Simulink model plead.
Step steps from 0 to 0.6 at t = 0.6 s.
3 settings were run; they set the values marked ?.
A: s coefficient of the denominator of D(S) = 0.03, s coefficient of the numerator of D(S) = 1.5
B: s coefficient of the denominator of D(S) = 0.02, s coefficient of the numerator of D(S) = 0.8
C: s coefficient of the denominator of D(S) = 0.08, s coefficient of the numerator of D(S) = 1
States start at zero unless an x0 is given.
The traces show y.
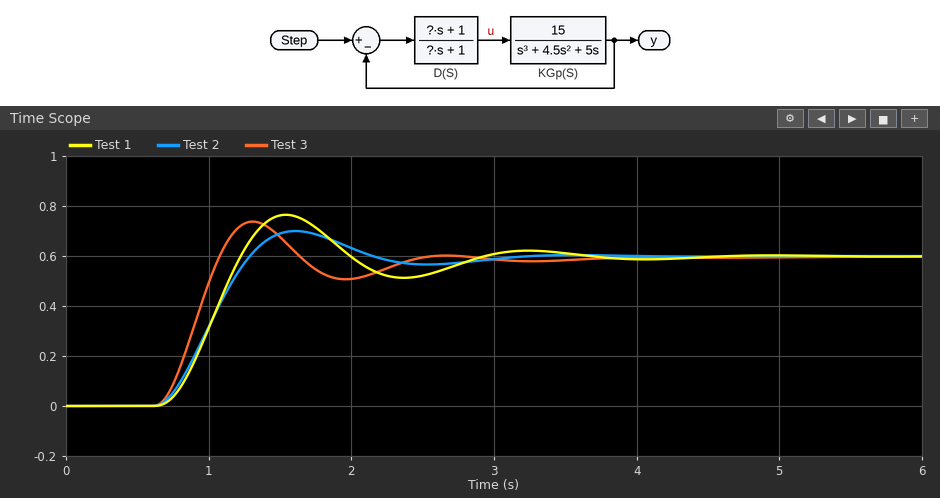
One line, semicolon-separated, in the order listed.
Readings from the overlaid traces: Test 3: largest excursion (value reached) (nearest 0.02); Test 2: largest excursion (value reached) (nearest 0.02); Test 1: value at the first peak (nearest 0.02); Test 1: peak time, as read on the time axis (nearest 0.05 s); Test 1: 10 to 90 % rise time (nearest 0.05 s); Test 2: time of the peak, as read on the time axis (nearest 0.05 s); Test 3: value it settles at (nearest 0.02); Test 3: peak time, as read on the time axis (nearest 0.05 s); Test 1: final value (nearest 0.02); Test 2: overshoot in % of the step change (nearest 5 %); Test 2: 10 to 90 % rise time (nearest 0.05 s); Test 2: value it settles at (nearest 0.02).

0.74; 0.70; 0.76; 1.55 s; 0.40 s; 1.60 s; 0.60; 1.30 s; 0.60; 15 %; 0.45 s; 0.60
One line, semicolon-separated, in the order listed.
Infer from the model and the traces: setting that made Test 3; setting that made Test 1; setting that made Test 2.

A; C; B
